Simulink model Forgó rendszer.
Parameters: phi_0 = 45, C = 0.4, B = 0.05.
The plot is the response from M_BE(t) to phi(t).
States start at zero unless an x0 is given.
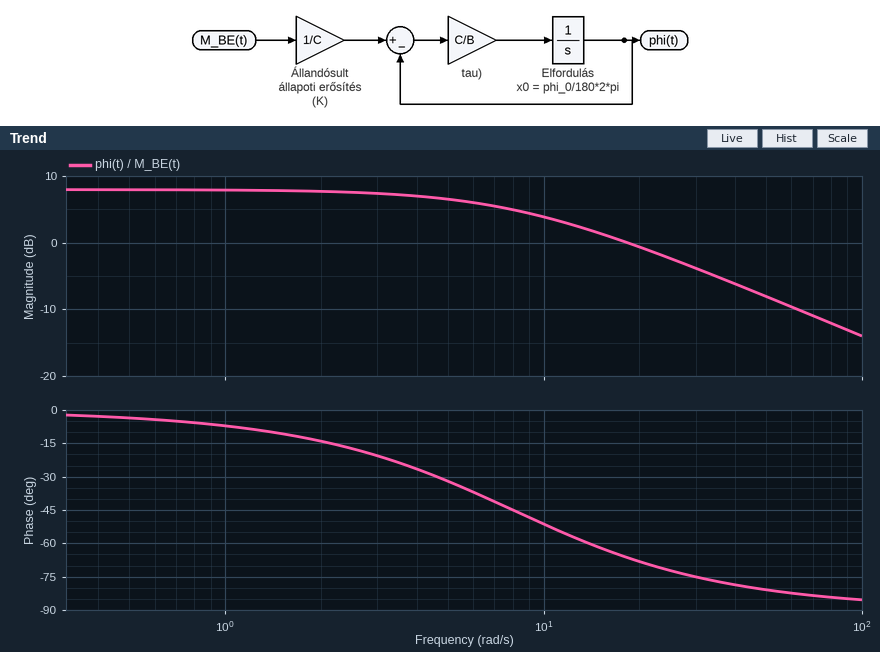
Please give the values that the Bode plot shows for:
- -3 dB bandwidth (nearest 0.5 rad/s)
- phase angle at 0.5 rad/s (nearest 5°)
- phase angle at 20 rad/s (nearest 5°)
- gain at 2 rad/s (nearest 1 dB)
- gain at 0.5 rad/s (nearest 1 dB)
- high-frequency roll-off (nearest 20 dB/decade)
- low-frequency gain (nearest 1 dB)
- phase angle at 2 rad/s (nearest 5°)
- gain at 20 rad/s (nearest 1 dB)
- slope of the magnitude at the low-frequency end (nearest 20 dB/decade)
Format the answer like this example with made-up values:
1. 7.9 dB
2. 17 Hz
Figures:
1. 8.0 rad/s
2. -5°
3. -70°
4. 8 dB
5. 8 dB
6. -20 dB/decade
7. 8 dB
8. -15°
9. -1 dB
10. 0 dB/decade
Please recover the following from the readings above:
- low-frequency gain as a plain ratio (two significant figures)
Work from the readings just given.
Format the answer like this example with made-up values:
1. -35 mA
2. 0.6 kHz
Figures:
1. 2.5
